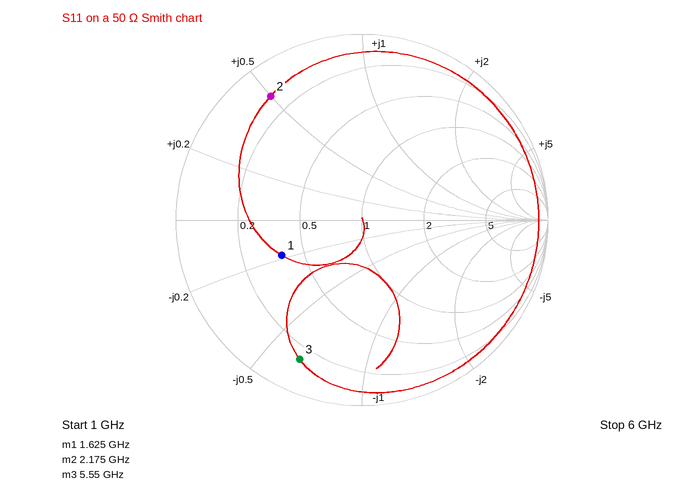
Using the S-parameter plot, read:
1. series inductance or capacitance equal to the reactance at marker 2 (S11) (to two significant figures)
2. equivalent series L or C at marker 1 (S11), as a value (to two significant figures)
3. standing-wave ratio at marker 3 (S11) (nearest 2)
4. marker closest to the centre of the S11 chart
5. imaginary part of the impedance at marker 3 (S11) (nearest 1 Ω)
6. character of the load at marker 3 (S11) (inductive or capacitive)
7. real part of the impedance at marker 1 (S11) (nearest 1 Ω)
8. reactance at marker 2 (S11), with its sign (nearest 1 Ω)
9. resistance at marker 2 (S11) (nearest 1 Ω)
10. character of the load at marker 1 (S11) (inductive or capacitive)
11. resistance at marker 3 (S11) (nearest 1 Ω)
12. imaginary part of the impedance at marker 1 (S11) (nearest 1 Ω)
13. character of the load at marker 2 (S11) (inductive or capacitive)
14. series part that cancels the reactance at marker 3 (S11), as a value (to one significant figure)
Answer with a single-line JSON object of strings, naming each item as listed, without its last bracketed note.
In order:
{"series inductance or capacitance equal to the reactance at marker 2 (S11)": "1.8 nH", "equivalent series L or C at marker 1 (S11), as a value": "11 pF", "standing-wave ratio at marker 3 (S11)": "10", "marker closest to the centre of the S11 chart": "marker 1", "imaginary part of the impedance at marker 3 (S11)": "-32 Ω", "character of the load at marker 3 (S11)": "capacitive", "real part of the impedance at marker 1 (S11)": "19 Ω", "reactance at marker 2 (S11), with its sign": "+25 Ω", "resistance at marker 2 (S11)": "6 Ω", "character of the load at marker 1 (S11)": "capacitive", "resistance at marker 3 (S11)": "7 Ω", "imaginary part of the impedance at marker 1 (S11)": "-9 Ω", "character of the load at marker 2 (S11)": "inductive", "series part that cancels the reactance at marker 3 (S11), as a value": "900 pH"}
